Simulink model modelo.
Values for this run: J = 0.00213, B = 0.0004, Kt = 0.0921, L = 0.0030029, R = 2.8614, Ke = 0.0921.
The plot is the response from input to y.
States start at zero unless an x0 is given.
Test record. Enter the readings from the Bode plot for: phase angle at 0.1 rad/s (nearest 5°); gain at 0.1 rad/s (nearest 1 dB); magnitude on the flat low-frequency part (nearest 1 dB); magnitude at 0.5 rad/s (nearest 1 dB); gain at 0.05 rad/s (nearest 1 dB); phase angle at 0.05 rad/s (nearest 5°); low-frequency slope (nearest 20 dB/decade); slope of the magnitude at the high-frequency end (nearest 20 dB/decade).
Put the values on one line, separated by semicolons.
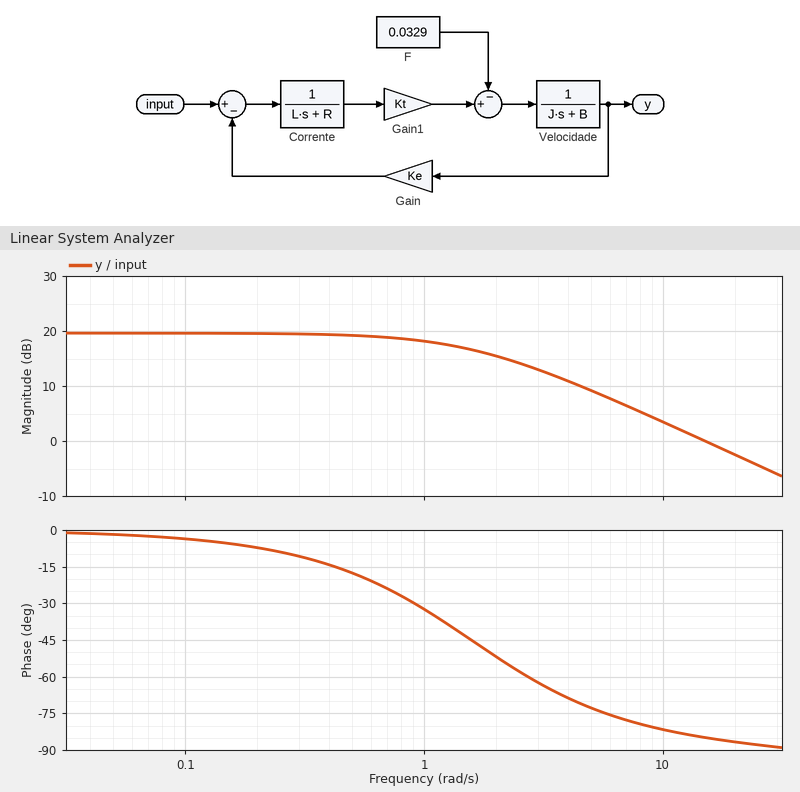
-5°; 20 dB; 20 dB; 19 dB; 20 dB; 0°; 0 dB/decade; -20 dB/decade
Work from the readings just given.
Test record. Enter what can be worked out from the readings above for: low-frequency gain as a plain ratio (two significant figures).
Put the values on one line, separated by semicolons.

10
